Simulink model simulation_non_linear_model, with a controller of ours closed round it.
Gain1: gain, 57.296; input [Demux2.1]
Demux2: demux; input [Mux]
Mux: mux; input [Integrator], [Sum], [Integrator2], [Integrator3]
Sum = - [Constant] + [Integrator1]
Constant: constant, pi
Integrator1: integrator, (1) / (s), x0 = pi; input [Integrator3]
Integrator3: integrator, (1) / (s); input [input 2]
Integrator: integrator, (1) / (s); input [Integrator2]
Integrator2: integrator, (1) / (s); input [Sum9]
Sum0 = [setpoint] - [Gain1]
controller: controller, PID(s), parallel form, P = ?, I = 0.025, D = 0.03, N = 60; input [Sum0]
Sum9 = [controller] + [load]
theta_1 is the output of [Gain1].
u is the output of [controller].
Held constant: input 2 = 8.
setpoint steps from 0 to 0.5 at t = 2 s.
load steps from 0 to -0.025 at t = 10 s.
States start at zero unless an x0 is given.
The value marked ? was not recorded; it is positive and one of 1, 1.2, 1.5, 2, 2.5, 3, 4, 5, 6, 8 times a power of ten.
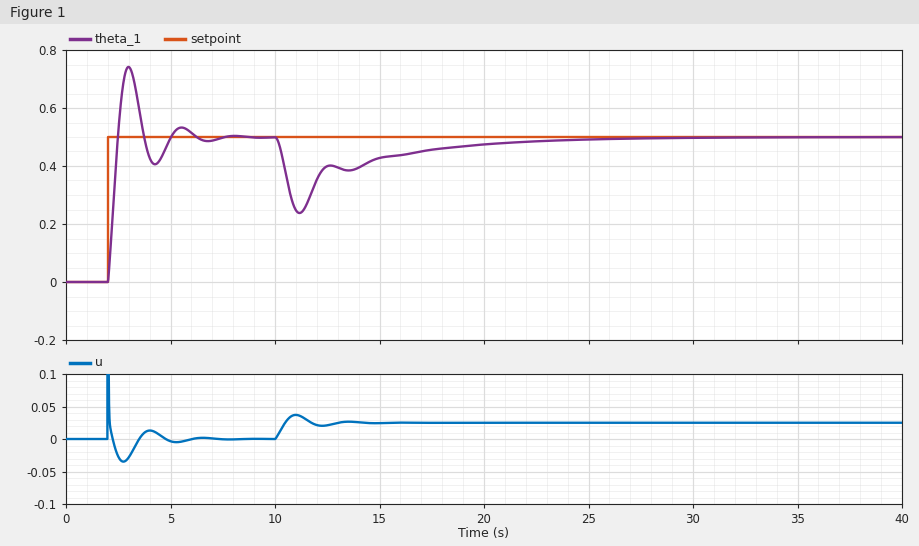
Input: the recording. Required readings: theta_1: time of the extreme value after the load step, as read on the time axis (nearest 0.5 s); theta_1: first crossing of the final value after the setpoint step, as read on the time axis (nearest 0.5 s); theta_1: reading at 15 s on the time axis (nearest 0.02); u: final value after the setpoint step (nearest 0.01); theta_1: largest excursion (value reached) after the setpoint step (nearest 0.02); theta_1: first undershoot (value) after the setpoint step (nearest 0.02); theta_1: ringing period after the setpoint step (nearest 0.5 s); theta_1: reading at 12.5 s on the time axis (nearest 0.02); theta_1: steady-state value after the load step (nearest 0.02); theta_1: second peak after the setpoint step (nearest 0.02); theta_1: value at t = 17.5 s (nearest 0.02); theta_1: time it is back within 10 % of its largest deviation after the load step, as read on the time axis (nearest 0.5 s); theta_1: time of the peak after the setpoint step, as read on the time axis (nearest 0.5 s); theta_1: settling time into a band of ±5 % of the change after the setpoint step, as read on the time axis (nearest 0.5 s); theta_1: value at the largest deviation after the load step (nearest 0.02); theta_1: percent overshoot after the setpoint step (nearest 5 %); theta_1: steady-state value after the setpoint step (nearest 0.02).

11.0 s
2.5 s
0.42
0.00
0.74
0.40
2.5 s
0.40
0.50
0.54
0.46
20.0 s
3.0 s
6.0 s
0.24
50 %
0.50
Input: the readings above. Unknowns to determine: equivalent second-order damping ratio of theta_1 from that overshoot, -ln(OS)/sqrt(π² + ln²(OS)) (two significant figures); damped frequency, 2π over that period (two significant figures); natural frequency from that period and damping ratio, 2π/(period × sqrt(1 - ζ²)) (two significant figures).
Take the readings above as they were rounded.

0.22
2.5 rad/s
2.6 rad/s
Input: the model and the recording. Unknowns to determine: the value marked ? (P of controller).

0.12
